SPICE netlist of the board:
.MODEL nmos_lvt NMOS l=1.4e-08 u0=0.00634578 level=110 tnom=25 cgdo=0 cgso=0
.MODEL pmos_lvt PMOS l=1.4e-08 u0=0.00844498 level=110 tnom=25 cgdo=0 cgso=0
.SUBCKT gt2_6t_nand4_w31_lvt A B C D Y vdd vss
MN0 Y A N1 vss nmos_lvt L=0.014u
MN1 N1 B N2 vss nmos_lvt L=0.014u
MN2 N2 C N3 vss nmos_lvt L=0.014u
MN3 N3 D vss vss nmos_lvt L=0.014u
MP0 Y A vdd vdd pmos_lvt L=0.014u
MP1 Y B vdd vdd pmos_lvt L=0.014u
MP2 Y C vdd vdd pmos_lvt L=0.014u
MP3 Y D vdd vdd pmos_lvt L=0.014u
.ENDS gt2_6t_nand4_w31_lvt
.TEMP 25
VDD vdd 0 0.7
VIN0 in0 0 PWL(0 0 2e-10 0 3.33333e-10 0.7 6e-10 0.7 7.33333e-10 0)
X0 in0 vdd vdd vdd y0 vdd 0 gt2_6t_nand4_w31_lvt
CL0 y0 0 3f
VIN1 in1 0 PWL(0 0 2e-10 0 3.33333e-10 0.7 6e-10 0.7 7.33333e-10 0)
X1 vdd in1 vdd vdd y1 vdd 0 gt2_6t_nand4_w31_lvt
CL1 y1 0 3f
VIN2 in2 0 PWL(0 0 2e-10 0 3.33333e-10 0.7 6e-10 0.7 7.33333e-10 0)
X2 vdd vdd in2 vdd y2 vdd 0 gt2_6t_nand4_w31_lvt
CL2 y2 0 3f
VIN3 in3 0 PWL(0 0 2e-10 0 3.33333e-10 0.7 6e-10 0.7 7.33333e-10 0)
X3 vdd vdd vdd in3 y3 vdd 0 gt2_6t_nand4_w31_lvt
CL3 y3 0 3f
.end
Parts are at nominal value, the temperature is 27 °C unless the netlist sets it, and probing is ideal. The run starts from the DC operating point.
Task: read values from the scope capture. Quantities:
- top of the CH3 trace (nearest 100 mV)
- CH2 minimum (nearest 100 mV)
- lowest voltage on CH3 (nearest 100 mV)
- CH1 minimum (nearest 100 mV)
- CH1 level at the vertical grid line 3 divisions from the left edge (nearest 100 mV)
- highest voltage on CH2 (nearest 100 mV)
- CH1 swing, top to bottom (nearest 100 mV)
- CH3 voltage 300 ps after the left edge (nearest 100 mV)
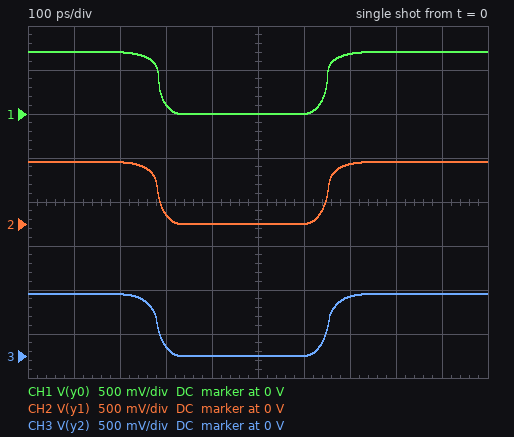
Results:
700 mV
0 V
0 V
0 V
100 mV
700 mV
700 mV
100 mV
